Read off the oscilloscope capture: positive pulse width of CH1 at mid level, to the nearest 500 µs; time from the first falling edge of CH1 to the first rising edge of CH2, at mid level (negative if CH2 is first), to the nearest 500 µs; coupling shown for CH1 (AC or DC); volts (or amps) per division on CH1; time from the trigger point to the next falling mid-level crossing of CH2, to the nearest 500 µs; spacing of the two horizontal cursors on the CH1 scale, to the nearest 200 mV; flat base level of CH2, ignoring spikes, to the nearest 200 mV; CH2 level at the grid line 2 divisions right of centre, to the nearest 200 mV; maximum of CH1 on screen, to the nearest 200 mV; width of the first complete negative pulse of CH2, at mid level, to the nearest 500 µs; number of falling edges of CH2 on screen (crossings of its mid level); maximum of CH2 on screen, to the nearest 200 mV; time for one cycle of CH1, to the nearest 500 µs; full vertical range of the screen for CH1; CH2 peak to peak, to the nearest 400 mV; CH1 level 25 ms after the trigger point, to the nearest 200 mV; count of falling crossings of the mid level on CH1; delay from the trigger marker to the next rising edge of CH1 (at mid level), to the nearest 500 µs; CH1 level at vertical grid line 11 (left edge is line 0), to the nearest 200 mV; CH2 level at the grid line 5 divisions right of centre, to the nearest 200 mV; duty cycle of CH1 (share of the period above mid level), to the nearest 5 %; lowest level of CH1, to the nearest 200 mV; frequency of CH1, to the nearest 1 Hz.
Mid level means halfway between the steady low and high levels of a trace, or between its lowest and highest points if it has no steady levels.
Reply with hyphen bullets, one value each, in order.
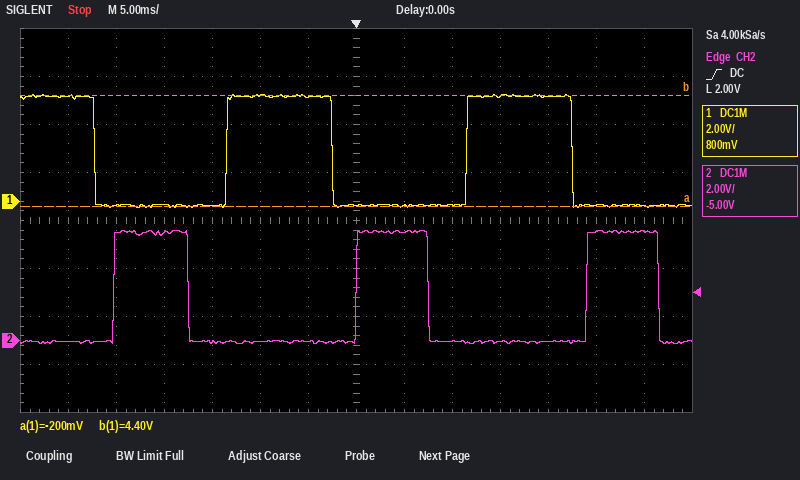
- 11.0 ms
- +2.0 ms
- DC
- 2 V
- 7.5 ms
- 4.6 V
- 0.0 V
- 0.0 V
- 4.4 V
- 17.5 ms
- 3
- 4.6 V
- 25.0 ms
- 16 V
- 4.8 V
- -200 mV
- 3
- 11.5 ms
- 4.4 V
- 4.6 V
- 45 %
- -200 mV
- 40 Hz
